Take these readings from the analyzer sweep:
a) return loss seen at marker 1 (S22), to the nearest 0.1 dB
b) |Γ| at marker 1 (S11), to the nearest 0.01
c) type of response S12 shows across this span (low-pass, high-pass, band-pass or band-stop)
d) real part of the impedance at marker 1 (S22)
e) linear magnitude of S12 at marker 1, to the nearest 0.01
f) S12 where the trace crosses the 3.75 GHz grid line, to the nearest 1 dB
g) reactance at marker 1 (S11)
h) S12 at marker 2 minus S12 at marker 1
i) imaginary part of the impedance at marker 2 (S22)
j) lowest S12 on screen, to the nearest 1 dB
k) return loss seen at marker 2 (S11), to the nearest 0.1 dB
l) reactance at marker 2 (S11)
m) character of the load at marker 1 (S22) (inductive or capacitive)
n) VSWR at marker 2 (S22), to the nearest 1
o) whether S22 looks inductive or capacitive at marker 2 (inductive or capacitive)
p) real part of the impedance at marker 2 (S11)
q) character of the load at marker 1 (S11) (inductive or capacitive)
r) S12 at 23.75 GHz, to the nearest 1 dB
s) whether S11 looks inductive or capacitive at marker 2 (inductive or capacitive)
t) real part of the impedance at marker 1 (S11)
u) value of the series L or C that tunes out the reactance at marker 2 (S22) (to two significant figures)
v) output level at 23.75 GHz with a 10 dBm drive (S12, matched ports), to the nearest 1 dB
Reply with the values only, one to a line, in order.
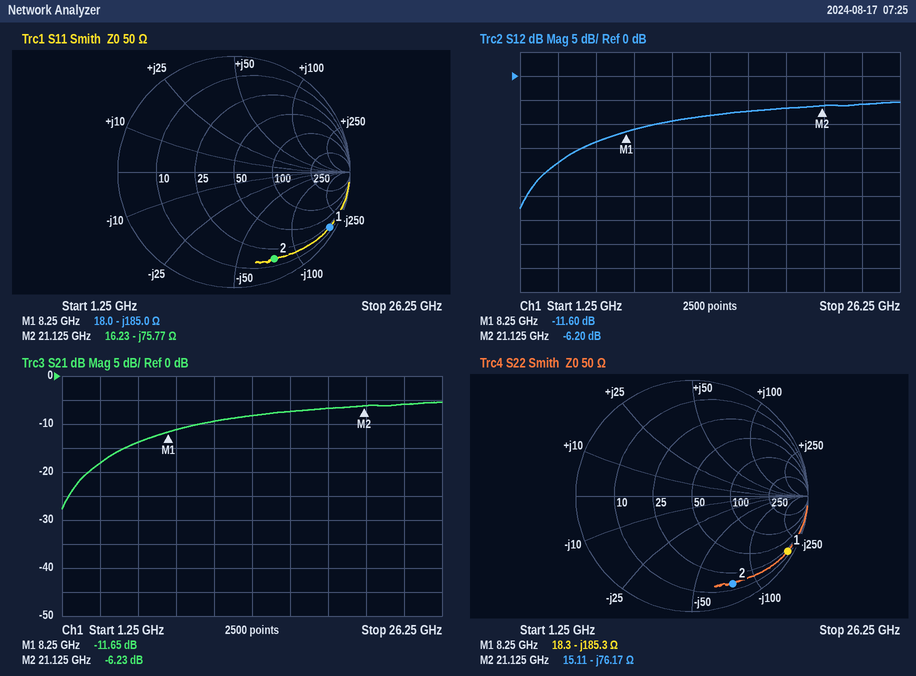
0.4 dB
0.95
high-pass
18.3 Ω
0.26
-18 dB
-185.0 Ω
5.40 dB
-76.17 Ω
-28 dB
1.7 dB
-75.77 Ω
capacitive
11
capacitive
16.23 Ω
capacitive
-6 dB
capacitive
18.0 Ω
570 pH
4 dBm
